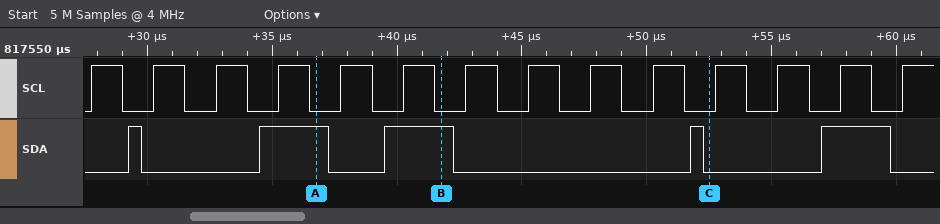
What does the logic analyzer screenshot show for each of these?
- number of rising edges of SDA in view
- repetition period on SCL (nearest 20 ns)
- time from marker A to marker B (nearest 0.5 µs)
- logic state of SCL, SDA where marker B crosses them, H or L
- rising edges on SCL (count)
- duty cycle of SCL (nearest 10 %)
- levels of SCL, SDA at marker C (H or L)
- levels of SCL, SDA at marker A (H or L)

5
2500 ns
5 µs
SCL=L, SDA=H
14
50 %
SCL=L, SDA=L
SCL=L, SDA=H
